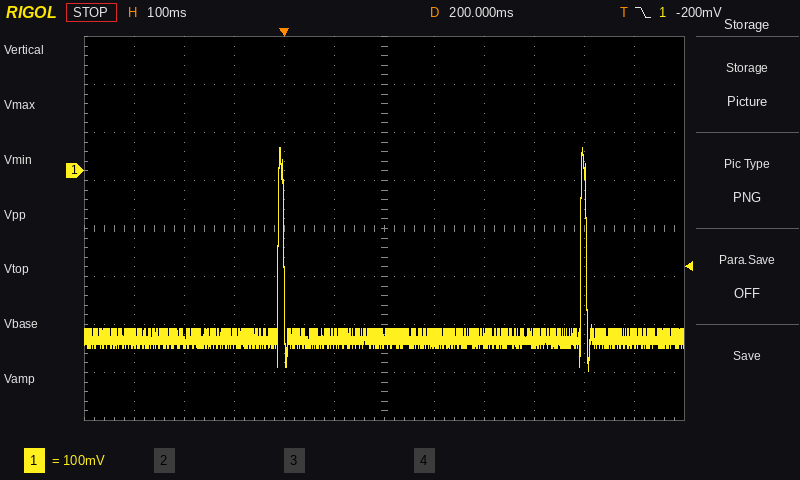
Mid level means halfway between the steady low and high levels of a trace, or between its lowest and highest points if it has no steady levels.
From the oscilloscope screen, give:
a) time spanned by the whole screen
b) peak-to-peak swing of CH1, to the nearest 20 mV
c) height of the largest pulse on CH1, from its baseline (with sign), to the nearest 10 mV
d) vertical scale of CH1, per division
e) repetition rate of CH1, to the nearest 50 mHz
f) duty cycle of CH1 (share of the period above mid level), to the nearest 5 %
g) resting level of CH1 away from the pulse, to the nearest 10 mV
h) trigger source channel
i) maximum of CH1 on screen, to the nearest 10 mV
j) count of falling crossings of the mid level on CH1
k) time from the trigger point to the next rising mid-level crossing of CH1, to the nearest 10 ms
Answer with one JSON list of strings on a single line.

["1.2 s", "460 mV", "+400 mV", "100 mV", "1.65 Hz", "0 %", "-350 mV", "CH1", "50 mV", "2", "590 ms"]
